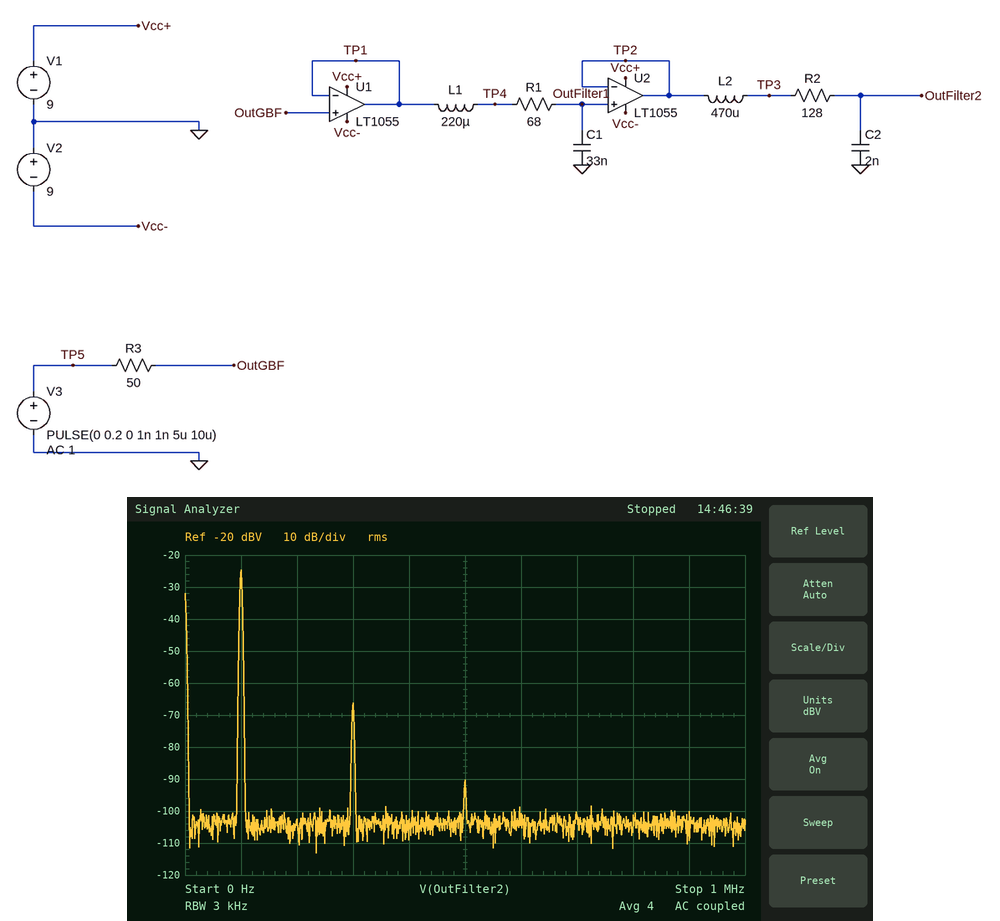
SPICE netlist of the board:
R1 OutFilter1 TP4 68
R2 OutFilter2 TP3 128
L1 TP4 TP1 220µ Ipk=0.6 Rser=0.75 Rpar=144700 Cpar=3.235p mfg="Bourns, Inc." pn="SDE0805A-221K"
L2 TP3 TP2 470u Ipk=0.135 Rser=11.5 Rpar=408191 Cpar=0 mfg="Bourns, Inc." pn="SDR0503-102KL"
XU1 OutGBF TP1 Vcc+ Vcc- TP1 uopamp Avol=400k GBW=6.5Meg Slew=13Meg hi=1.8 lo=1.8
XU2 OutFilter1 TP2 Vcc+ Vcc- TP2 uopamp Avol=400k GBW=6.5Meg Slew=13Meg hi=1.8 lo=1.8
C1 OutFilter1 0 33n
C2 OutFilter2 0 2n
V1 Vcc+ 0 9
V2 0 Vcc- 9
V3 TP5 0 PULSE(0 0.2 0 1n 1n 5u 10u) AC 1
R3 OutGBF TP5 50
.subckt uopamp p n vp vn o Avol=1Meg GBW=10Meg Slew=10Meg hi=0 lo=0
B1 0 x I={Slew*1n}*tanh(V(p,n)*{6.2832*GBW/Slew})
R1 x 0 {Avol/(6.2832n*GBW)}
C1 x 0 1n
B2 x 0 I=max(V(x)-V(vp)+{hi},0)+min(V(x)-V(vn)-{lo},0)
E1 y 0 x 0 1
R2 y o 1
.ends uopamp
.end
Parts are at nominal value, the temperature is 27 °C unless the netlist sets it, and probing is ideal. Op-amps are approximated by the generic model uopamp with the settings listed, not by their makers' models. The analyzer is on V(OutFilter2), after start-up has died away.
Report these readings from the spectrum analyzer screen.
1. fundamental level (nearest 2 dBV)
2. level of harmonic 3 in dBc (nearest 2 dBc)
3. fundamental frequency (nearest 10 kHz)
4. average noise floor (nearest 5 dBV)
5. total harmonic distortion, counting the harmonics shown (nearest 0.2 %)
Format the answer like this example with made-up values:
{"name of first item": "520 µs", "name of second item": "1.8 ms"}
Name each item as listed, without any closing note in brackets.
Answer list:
{"fundamental level": "-24 dBV", "level of harmonic 3 in dBc": "-42 dBc", "fundamental frequency": "100 kHz", "average noise floor": "-105 dBV", "total harmonic distortion, counting the harmonics shown": "0.8 %"}
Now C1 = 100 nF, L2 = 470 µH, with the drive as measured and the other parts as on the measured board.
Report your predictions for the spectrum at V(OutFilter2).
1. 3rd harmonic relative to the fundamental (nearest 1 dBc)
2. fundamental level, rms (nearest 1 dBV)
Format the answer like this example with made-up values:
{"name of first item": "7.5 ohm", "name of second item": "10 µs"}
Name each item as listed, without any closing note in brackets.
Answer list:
{"3rd harmonic relative to the fundamental": "-40 dBc", "fundamental level, rms": "-36 dBV"}
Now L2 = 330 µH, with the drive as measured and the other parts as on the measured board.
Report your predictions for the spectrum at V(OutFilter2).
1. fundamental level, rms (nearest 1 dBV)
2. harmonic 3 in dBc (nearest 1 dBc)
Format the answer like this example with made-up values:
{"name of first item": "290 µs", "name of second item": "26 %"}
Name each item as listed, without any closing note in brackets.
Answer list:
{"fundamental level, rms": "-26 dBV", "harmonic 3 in dBc": "-36 dBc"}
